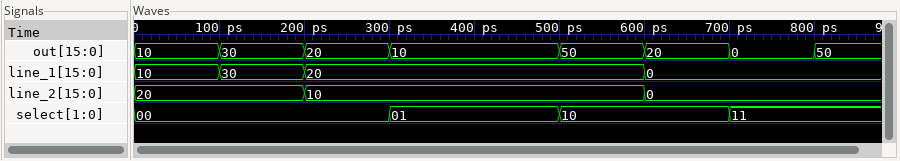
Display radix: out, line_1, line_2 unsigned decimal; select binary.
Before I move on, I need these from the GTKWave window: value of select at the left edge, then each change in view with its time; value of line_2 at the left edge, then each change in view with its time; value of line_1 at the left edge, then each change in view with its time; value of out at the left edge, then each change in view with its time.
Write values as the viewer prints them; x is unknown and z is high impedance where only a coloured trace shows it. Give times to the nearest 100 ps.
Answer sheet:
00, 01 at 300 ps, 10 at 500 ps, 11 at 700 ps
20, 10 at 200 ps, 0 at 600 ps
10, 30 at 100 ps, 20 at 200 ps, 0 at 600 ps
10, 30 at 100 ps, 20 at 200 ps, 10 at 300 ps, 50 at 500 ps, 20 at 600 ps, 0 at 700 ps, 50 at 800 ps
